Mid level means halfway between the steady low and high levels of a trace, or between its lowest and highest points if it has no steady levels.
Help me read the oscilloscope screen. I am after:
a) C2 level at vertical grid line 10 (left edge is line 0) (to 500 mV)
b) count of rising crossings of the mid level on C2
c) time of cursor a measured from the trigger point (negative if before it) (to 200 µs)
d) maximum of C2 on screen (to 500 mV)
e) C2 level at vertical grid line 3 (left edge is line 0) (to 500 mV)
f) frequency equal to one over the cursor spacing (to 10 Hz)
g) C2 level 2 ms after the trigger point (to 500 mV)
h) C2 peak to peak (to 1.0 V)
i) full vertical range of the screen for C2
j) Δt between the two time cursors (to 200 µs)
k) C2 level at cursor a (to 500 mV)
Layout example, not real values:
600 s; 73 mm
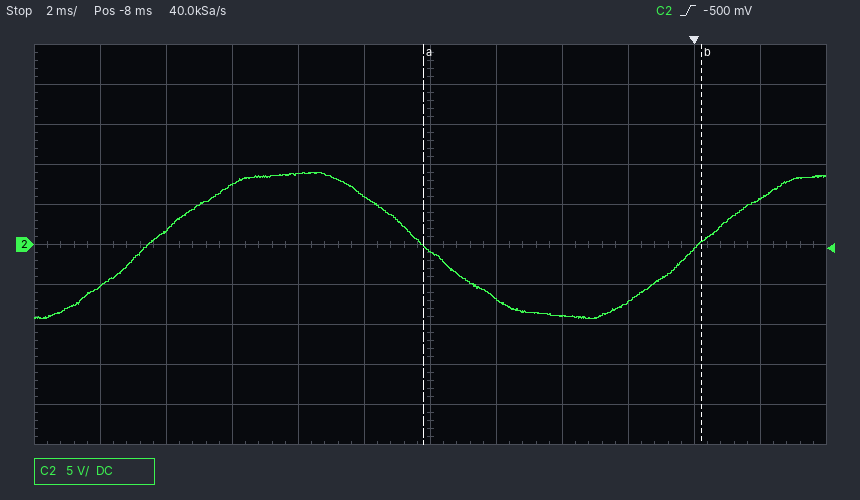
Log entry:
-500 mV; 2; -8.2 ms; 9.0 V; 7.5 V; 120 Hz; 5.5 V; 18.0 V; 50 V; 8.4 ms; 0.0 V
